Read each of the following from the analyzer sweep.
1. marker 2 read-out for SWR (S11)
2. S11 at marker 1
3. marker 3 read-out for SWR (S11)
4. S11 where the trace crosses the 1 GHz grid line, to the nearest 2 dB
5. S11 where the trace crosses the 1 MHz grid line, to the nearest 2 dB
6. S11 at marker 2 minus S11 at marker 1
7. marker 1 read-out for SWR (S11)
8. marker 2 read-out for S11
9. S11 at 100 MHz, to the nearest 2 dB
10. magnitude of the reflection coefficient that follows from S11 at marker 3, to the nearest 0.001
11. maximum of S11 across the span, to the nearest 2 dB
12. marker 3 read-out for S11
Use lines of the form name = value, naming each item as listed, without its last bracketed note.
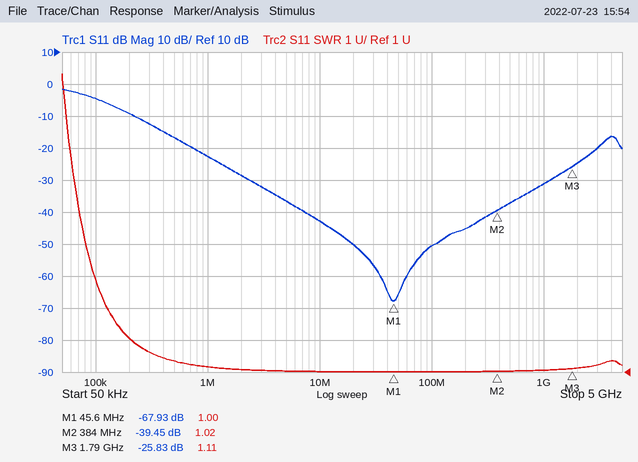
marker 2 read-out for SWR = 1.02
S11 at marker 1 = -67.93 dB
marker 3 read-out for SWR = 1.11
S11 where the trace crosses the 1 GHz grid line, to the nearest 2 dB = -32 dB
S11 where the trace crosses the 1 MHz grid line, to the nearest 2 dB = -22 dB
S11 at marker 2 minus S11 at marker 1 = 28.48 dB
marker 1 read-out for SWR = 1.00
marker 2 read-out for S11 = -39.45 dB
S11 at 100 MHz, to the nearest 2 dB = -50 dB
magnitude of the reflection coefficient that follows from S11 at marker 3, to the nearest 0.001 = 0.051
maximum of S11 across the span, to the nearest 2 dB = -2 dB
marker 3 read-out for S11 = -25.83 dB
